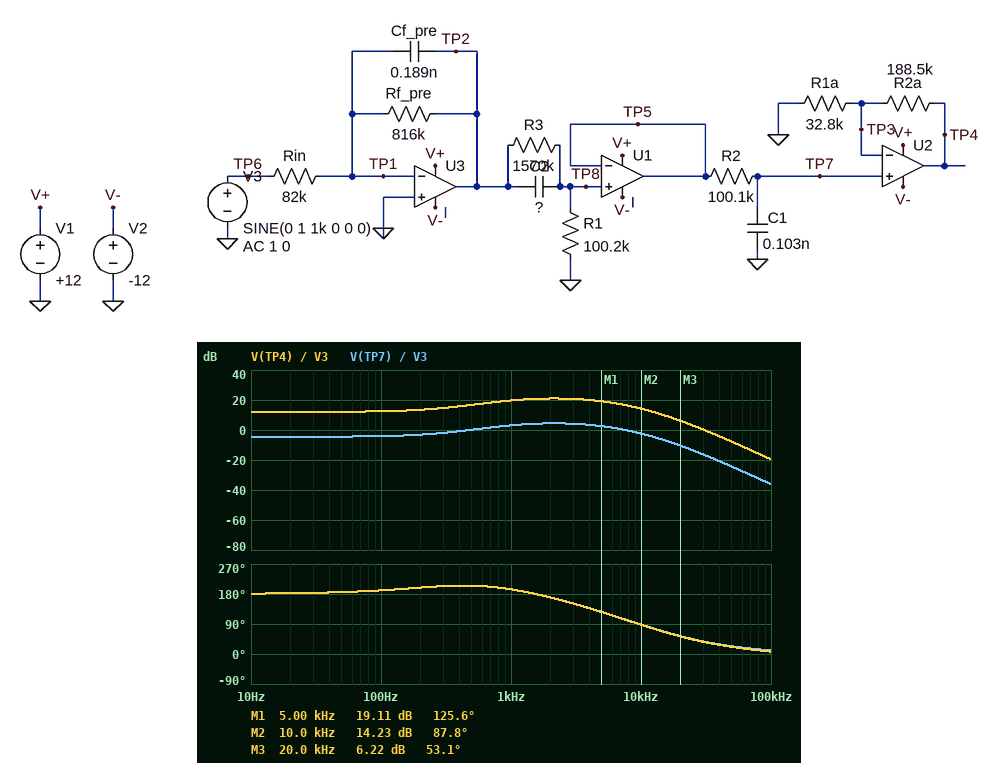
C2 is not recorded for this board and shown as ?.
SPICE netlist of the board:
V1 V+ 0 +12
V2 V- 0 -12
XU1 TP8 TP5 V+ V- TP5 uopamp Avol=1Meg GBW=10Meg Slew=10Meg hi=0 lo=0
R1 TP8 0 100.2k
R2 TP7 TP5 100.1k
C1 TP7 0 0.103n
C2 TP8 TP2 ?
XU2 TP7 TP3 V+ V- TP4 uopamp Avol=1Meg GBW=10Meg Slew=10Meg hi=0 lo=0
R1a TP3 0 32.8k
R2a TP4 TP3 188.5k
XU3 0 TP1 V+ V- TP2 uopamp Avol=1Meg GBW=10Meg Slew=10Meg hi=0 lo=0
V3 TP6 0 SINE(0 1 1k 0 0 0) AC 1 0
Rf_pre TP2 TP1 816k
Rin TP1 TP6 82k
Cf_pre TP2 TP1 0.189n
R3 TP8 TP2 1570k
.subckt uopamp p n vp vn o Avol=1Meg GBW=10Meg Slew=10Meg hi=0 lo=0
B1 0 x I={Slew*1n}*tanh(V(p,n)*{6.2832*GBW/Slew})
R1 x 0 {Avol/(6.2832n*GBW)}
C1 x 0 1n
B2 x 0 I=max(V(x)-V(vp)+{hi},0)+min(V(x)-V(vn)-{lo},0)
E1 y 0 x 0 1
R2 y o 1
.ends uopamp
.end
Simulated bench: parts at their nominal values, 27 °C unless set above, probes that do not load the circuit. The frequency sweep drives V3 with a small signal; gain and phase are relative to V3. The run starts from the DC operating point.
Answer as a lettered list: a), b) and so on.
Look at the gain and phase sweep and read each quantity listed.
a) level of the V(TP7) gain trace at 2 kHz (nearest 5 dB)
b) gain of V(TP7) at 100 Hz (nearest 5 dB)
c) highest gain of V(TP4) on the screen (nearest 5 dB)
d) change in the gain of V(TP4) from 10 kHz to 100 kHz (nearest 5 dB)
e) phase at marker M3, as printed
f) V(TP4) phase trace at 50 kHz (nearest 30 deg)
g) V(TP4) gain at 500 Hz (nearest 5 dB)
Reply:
a) 5 dB
b) -5 dB
c) 20 dB
d) -35 dB
e) 53.1 deg
f) 30 deg
g) 15 dB
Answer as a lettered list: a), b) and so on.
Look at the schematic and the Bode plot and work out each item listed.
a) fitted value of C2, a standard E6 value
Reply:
a) 330 pF
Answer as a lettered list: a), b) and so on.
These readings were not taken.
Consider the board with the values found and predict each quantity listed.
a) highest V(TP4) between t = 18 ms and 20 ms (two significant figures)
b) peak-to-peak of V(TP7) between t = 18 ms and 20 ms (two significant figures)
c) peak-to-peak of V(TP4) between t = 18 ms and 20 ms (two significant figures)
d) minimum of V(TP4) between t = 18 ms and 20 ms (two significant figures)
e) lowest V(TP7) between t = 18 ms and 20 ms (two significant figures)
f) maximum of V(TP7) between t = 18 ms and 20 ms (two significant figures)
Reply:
a) 9.6 V
b) 2.9 V
c) 19 V
d) -9.6 V
e) -1.4 V
f) 1.4 V
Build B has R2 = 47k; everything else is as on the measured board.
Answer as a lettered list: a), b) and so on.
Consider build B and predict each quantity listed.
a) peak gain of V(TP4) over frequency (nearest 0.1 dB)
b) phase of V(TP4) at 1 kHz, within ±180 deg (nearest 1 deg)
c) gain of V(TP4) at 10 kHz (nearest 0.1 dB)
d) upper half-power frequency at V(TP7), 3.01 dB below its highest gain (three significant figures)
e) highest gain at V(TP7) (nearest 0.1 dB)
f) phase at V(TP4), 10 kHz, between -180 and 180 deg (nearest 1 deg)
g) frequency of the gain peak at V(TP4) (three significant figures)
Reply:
a) 21.1 dB
b) -164 deg
c) 15.4 dB
d) 6.63 kHz
e) 4.5 dB
f) 104 deg
g) 2.20 kHz
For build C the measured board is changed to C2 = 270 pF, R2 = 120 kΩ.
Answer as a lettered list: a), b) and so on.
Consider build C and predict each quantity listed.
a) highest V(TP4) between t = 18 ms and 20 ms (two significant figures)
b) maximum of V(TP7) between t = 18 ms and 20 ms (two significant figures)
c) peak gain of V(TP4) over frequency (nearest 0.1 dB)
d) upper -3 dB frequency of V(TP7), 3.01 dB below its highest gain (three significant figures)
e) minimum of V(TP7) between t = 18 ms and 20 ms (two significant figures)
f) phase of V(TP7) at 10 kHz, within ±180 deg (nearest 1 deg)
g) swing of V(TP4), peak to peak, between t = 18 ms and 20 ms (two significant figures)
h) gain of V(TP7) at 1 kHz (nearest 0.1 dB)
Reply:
a) 8.1 V
b) 1.2 V
c) 19.5 dB
d) 6.63 kHz
e) -1.2 V
f) 88 deg
g) 16 V
h) 1.6 dB
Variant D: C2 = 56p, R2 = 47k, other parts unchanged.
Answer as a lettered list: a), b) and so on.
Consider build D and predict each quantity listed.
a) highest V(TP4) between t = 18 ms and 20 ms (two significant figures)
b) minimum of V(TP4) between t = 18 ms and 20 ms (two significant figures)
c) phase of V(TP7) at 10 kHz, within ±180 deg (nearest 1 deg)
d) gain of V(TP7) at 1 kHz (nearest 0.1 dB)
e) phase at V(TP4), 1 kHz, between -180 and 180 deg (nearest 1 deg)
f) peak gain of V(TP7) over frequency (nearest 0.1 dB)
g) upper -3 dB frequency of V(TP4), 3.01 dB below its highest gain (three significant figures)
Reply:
a) 3.3 V
b) -3.3 V
c) 140 deg
d) -6.2 dB
e) 161 deg
f) -4.5 dB
g) 1.72 kHz
